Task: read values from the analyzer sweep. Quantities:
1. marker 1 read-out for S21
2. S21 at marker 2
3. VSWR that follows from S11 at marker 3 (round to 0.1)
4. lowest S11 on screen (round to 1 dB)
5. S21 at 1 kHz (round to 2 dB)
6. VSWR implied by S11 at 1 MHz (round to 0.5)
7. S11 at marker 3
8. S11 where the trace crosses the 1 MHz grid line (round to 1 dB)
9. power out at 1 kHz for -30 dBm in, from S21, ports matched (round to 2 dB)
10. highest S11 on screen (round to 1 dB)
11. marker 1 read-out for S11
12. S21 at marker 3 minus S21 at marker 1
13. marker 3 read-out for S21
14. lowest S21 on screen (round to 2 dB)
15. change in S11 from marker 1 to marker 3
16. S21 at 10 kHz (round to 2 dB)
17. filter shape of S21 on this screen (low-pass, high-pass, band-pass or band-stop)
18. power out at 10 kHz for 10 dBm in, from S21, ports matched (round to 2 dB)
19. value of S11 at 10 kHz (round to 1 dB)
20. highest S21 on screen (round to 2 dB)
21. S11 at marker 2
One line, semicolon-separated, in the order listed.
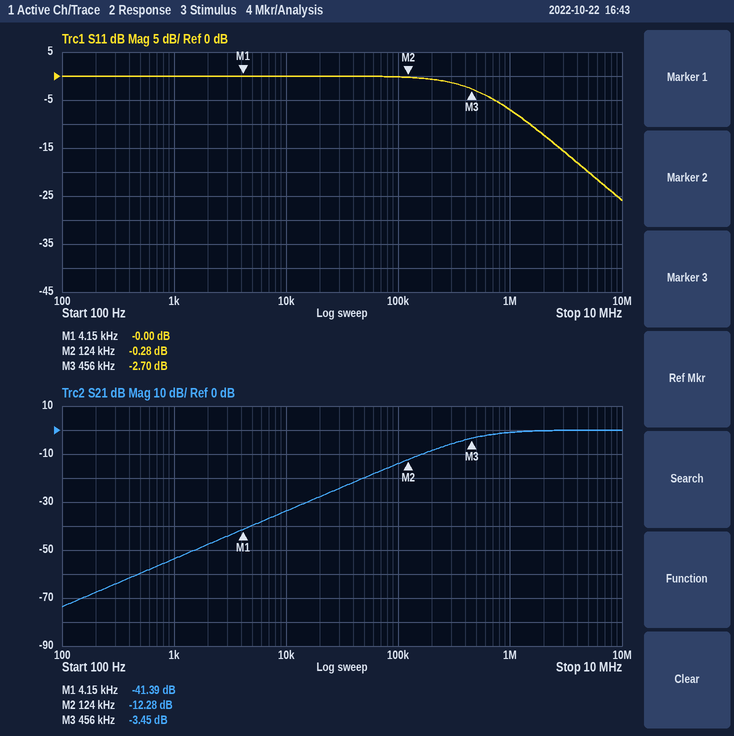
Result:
-41.39 dB; -12.28 dB; 6.5; -26 dB; -54 dB; 2.5; -2.70 dB; -7 dB; -84 dBm; 0 dB; -0.00 dB; 37.94 dB; -3.45 dB; -74 dB; -2.70 dB; -34 dB; high-pass; -24 dBm; 0 dB; 0 dB; -0.28 dB
